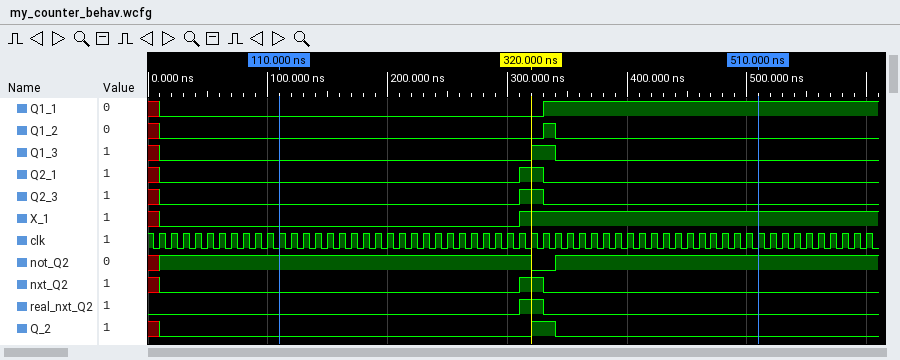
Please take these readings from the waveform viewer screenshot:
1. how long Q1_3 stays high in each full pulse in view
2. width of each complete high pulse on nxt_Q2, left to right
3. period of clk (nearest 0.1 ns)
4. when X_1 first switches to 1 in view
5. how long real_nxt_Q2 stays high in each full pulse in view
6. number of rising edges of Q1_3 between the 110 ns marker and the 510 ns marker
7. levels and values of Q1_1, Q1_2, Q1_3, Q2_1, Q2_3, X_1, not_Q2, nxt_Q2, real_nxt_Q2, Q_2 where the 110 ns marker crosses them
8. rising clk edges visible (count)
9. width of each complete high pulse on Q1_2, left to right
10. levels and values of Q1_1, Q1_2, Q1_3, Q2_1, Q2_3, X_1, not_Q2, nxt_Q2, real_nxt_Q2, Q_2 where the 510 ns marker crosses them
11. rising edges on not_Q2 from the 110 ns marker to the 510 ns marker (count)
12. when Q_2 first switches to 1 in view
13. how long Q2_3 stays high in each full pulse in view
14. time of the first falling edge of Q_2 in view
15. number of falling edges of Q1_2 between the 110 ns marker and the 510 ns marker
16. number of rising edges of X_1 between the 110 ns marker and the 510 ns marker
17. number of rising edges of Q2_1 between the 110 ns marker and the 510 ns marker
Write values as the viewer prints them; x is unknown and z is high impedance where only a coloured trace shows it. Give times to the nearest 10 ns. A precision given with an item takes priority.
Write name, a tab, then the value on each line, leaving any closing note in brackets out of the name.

how long Q1_3 stays high in each full pulse in view	20 ns
width of each complete high pulse on nxt_Q2, left to right	20 ns
period of clk	10 ns
when X_1 first switches to 1 in view	310 ns
how long real_nxt_Q2 stays high in each full pulse in view	20 ns
number of rising edges of Q1_3 between the 110 ns marker and the 510 ns marker	1
levels and values of Q1_1, Q1_2, Q1_3, Q2_1, Q2_3, X_1, not_Q2, nxt_Q2, real_nxt_Q2, Q_2 where the 110 ns marker crosses them	Q1_1=0, Q1_2=0, Q1_3=0, Q2_1=0, Q2_3=0, X_1=0, not_Q2=1, nxt_Q2=0, real_nxt_Q2=0, Q_2=0
rising clk edges visible	60
width of each complete high pulse on Q1_2, left to right	10 ns
levels and values of Q1_1, Q1_2, Q1_3, Q2_1, Q2_3, X_1, not_Q2, nxt_Q2, real_nxt_Q2, Q_2 where the 510 ns marker crosses them	Q1_1=1, Q1_2=0, Q1_3=0, Q2_1=0, Q2_3=0, X_1=1, not_Q2=1, nxt_Q2=0, real_nxt_Q2=0, Q_2=0
rising edges on not_Q2 from the 110 ns marker to the 510 ns marker	1
when Q_2 first switches to 1 in view	320 ns
how long Q2_3 stays high in each full pulse in view	20 ns
time of the first falling edge of Q_2 in view	340 ns
number of falling edges of Q1_2 between the 110 ns marker and the 510 ns marker	1
number of rising edges of X_1 between the 110 ns marker and the 510 ns marker	1
number of rising edges of Q2_1 between the 110 ns marker and the 510 ns marker	1
